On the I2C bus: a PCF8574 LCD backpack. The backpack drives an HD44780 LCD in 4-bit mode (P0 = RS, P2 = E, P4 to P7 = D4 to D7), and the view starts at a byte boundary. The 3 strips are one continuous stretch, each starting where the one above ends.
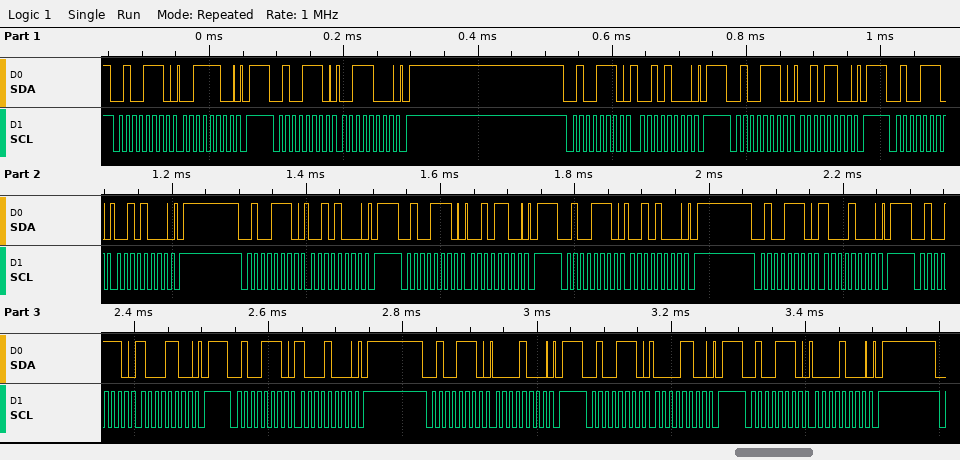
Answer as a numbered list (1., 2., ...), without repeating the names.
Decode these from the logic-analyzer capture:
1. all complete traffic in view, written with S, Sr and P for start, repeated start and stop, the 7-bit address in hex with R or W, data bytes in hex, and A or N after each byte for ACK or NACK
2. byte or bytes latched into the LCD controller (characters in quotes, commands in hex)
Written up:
1. S 27W A 3C A P S 27W A 38 A P S 27W A 28 A P S 27W A 2C A P S 27W A 28 A P S 27W A 28 A P S 27W A 2C A P S 27W A 28 A P S 27W A 88 A P S 27W A 8C A P S 27W A 88 A P S 27W A 08 A P S 27W A 0C A P S 27W A 08 A P
2. 0x28
